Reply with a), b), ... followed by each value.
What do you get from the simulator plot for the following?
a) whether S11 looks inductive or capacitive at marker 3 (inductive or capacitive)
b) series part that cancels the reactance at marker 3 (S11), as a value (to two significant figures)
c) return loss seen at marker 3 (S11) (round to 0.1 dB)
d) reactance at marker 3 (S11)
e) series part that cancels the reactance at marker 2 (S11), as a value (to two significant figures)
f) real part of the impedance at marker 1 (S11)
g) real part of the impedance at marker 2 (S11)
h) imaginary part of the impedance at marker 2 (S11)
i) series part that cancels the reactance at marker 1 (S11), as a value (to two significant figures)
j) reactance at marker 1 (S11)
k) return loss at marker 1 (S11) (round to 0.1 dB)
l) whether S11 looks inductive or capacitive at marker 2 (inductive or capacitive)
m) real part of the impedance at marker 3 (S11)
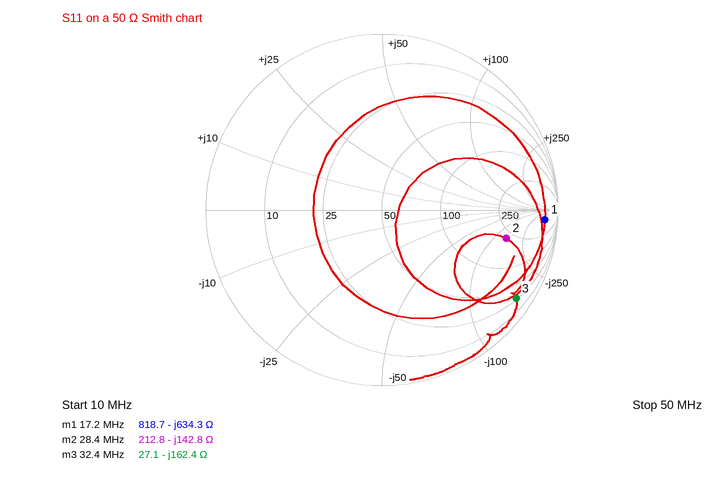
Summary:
a) capacitive
b) 800 nH
c) 0.8 dB
d) -162.4 Ω
e) 800 nH
f) 818.7 Ω
g) 212.8 Ω
h) -142.8 Ω
i) 5.9 µH
j) -634.3 Ω
k) 0.7 dB
l) capacitive
m) 27.1 Ω
